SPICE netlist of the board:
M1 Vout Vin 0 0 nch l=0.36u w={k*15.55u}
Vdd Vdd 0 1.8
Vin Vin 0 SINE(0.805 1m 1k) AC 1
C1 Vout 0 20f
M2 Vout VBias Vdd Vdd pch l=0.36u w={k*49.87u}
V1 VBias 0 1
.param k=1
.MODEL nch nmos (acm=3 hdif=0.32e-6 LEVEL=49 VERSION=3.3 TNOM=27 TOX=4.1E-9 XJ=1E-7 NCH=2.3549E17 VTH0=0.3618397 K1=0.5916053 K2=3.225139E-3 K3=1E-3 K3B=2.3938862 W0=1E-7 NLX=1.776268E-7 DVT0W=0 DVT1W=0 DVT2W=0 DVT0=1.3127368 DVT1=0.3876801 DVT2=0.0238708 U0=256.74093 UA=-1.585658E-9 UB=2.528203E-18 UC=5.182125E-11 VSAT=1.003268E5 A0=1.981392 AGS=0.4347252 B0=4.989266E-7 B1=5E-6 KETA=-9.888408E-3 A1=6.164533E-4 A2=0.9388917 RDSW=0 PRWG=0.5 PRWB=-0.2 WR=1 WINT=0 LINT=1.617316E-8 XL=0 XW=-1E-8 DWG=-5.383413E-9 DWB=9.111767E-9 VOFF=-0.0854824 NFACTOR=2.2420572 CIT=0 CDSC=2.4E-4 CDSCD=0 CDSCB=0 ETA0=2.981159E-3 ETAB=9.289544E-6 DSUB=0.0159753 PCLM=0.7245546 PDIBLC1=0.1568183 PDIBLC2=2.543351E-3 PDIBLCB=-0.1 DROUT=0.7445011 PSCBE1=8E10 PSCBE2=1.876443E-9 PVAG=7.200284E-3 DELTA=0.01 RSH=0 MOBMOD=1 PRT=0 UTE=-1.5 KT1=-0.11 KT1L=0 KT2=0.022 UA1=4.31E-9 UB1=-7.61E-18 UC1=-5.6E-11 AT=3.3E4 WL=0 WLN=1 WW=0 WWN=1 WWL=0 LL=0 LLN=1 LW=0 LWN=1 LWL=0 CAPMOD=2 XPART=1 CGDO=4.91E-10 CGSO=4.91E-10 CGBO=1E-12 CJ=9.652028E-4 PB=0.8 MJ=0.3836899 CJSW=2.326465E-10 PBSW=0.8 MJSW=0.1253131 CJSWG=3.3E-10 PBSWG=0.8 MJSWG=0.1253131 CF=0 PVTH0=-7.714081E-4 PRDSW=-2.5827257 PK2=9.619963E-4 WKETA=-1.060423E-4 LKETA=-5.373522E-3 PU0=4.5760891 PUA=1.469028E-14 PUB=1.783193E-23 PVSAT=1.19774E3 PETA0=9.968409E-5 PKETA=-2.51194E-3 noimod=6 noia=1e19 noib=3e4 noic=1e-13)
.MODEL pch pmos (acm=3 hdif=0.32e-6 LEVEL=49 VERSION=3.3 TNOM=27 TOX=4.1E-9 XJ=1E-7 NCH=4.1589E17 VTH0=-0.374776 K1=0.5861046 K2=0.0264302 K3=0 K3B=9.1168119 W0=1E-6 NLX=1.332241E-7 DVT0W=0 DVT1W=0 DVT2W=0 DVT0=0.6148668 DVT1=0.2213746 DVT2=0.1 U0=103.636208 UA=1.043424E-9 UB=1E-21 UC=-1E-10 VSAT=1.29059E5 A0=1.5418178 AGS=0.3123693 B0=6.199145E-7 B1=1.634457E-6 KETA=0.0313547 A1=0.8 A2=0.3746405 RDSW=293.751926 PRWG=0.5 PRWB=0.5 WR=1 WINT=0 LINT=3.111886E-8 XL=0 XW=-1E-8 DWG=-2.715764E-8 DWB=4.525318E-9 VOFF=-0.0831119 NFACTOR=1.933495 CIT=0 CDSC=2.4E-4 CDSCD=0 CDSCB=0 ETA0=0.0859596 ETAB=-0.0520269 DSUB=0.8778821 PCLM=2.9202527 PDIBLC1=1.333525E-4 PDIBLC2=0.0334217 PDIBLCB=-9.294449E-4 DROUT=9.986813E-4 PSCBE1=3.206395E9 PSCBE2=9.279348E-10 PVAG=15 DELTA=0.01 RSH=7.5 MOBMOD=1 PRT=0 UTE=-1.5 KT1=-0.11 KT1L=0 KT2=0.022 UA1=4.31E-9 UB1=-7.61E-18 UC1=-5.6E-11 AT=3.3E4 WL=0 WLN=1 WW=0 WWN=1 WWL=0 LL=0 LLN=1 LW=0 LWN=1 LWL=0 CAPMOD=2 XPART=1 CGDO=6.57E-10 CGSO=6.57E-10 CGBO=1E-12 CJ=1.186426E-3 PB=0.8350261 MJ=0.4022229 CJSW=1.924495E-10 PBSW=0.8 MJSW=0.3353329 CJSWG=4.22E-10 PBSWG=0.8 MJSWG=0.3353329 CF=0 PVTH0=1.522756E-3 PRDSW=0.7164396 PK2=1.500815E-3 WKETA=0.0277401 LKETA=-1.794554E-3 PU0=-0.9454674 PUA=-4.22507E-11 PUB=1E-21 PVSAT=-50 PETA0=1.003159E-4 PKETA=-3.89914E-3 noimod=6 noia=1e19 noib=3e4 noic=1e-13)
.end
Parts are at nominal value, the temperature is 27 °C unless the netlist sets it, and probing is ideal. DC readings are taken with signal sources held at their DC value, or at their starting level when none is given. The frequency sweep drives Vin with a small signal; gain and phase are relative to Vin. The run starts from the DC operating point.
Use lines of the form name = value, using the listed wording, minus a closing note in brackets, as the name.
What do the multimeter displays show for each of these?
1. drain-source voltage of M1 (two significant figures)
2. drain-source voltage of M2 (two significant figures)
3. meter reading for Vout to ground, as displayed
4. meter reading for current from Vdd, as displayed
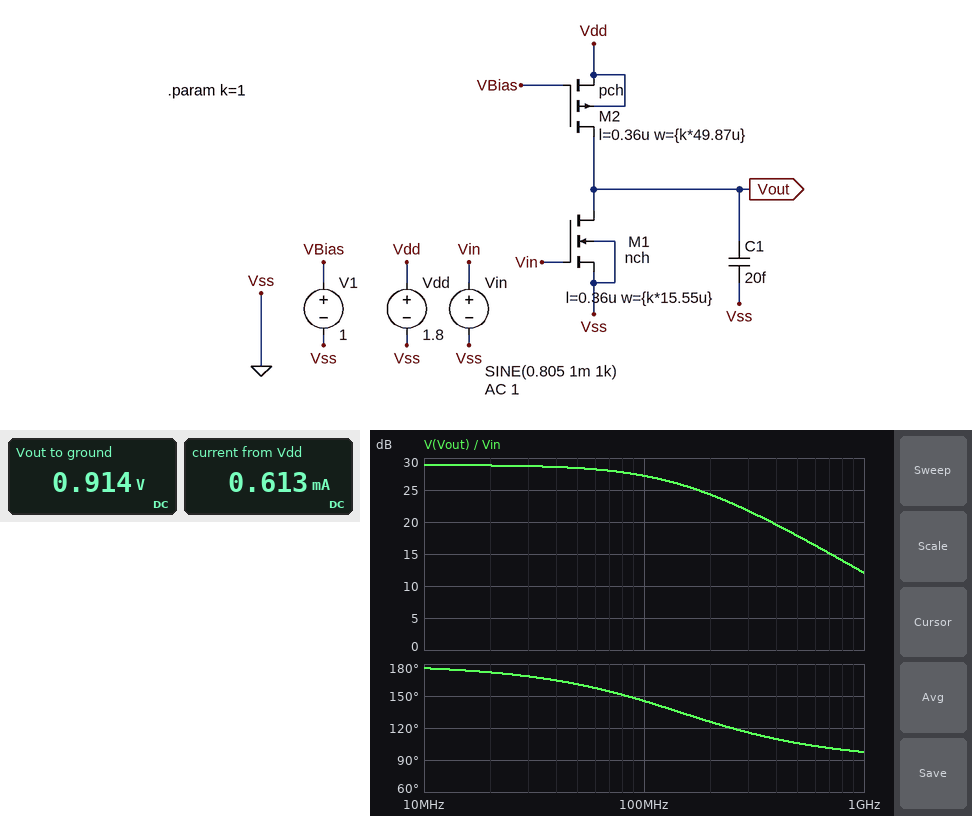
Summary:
drain-source voltage of M1 = 910 mV
drain-source voltage of M2 = -890 mV
meter reading for Vout to ground, as displayed = 0.914 V
meter reading for current from Vdd, as displayed = 0.613 mA
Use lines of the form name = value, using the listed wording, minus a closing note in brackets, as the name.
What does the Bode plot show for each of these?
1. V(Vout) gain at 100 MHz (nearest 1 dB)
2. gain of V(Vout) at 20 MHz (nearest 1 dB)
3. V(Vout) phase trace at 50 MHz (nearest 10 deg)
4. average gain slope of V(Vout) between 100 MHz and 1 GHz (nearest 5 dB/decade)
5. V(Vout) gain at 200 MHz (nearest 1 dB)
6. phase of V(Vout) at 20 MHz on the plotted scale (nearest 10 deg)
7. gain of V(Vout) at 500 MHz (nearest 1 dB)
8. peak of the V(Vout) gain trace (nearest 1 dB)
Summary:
V(Vout) gain at 100 MHz = 27 dB
gain of V(Vout) at 20 MHz = 29 dB
V(Vout) phase trace at 50 MHz = 160 deg
average gain slope of V(Vout) between 100 MHz and 1 GHz = -15 dB/decade
V(Vout) gain at 200 MHz = 24 dB
phase of V(Vout) at 20 MHz on the plotted scale = 170 deg
gain of V(Vout) at 500 MHz = 18 dB
peak of the V(Vout) gain trace = 29 dB
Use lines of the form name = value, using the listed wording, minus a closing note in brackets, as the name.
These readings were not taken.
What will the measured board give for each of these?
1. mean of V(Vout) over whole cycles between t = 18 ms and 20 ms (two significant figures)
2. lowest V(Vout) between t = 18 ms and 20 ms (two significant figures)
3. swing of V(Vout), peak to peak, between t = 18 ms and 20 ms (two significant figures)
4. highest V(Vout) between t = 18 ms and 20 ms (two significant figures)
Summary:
mean of V(Vout) over whole cycles between t = 18 ms and 20 ms = 910 mV
lowest V(Vout) between t = 18 ms and 20 ms = 890 mV
swing of V(Vout), peak to peak, between t = 18 ms and 20 ms = 56 mV
highest V(Vout) between t = 18 ms and 20 ms = 940 mV
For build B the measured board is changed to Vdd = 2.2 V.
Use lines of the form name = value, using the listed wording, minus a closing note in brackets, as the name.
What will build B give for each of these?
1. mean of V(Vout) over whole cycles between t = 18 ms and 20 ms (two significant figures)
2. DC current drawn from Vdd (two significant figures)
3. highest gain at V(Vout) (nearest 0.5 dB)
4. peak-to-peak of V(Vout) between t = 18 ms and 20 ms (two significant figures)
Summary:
mean of V(Vout) over whole cycles between t = 18 ms and 20 ms = 2.1 V
DC current drawn from Vdd = 660 µA
highest gain at V(Vout) = -5.0 dB
peak-to-peak of V(Vout) between t = 18 ms and 20 ms = 1.1 mV
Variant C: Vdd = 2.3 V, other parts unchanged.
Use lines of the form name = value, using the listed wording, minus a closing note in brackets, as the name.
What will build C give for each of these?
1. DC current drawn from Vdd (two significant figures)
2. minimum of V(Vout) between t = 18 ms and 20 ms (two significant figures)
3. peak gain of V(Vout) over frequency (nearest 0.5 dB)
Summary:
DC current drawn from Vdd = 670 µA
minimum of V(Vout) between t = 18 ms and 20 ms = 2.2 V
peak gain of V(Vout) over frequency = -6.0 dB
